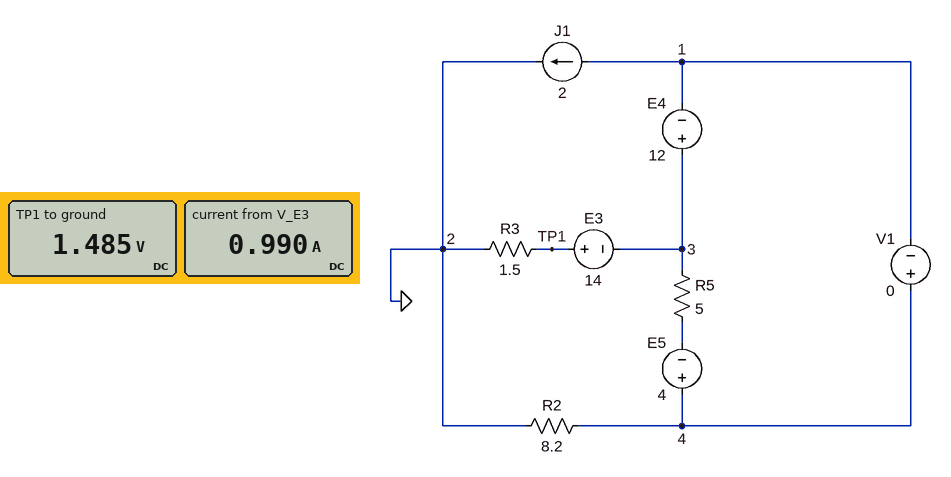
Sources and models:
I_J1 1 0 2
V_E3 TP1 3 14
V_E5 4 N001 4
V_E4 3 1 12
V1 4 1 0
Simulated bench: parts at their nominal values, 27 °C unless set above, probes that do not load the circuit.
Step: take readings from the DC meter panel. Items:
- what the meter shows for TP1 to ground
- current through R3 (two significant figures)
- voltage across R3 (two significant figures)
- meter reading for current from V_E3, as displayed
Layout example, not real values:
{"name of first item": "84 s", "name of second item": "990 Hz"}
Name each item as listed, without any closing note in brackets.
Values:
{"what the meter shows for TP1 to ground": "1.485 V", "current through R3": "990 mA", "voltage across R3": "1.5 V", "meter reading for current from V_E3, as displayed": "0.990 A"}
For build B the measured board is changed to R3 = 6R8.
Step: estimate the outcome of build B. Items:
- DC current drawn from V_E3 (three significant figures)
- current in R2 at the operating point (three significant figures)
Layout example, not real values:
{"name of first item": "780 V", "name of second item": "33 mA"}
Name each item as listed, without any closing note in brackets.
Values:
{"DC current drawn from V_E3": "640 mA", "current in R2 at the operating point": "2.64 A"}
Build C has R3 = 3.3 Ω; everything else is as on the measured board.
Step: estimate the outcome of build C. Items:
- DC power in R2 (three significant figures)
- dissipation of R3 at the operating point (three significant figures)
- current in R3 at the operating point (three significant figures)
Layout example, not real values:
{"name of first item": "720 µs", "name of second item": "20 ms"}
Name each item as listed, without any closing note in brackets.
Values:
{"DC power in R2": "65.9 W", "dissipation of R3 at the operating point": "2.30 W", "current in R3 at the operating point": "835 mA"}
